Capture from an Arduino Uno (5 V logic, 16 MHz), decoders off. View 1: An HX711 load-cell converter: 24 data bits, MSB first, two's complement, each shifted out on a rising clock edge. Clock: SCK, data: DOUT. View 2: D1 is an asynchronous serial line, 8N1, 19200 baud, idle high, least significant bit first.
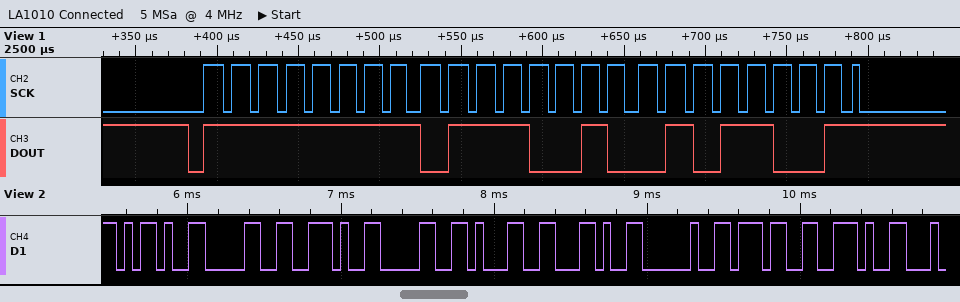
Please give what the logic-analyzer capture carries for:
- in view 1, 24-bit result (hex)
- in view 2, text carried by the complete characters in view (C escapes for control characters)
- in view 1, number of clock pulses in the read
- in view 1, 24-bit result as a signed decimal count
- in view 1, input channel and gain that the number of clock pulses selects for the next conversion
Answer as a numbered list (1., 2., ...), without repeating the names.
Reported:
1. 0xFF7259
2. "-0.01, 7."
3. 25
4. -36263
5. channel A, gain 128
